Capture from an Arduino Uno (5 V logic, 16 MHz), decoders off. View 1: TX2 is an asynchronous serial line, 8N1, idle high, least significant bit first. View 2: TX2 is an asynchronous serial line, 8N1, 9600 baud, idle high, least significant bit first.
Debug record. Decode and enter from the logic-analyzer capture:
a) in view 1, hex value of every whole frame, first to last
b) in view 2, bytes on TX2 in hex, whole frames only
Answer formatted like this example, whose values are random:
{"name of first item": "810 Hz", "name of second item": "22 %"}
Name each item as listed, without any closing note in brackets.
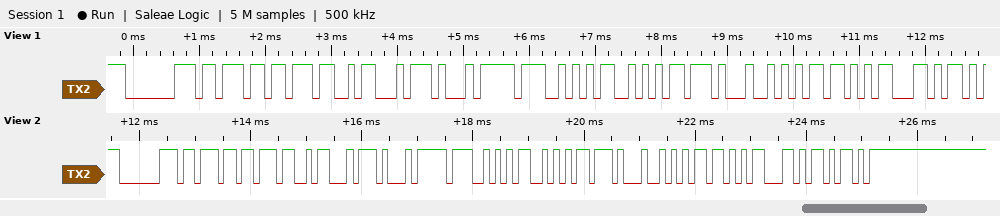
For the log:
{"in view 1, hex value of every whole frame, first to last": "C0 BB BB 1A 17 DF AA AA 17 AA AB AC", "in view 2, bytes on TX2 in hex, whole frames only": "0xC0 0xBB 0xBB 0x1A 0x17 0xDF 0xAA 0xAA 0x17 0xAA 0xAB 0xAC 0xAD"}
